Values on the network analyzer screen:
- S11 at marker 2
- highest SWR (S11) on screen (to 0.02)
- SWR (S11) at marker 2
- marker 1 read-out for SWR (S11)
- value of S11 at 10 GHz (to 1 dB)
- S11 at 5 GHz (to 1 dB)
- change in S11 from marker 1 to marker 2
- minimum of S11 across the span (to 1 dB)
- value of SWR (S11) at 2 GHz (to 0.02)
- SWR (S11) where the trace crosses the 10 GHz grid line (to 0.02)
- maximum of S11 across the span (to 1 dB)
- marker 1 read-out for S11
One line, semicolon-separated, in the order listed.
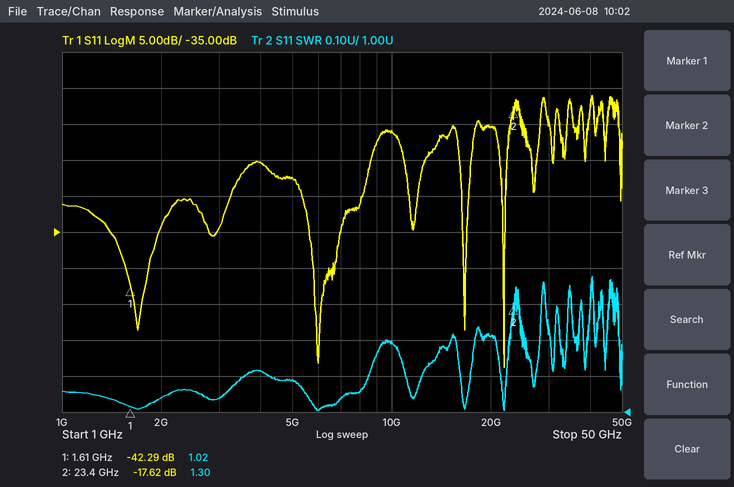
-17.62 dB; 1.38; 1.30; 1.02; -21 dB; -27 dB; 24.67 dB; -54 dB; 1.04; 1.20; -16 dB; -42.29 dB
